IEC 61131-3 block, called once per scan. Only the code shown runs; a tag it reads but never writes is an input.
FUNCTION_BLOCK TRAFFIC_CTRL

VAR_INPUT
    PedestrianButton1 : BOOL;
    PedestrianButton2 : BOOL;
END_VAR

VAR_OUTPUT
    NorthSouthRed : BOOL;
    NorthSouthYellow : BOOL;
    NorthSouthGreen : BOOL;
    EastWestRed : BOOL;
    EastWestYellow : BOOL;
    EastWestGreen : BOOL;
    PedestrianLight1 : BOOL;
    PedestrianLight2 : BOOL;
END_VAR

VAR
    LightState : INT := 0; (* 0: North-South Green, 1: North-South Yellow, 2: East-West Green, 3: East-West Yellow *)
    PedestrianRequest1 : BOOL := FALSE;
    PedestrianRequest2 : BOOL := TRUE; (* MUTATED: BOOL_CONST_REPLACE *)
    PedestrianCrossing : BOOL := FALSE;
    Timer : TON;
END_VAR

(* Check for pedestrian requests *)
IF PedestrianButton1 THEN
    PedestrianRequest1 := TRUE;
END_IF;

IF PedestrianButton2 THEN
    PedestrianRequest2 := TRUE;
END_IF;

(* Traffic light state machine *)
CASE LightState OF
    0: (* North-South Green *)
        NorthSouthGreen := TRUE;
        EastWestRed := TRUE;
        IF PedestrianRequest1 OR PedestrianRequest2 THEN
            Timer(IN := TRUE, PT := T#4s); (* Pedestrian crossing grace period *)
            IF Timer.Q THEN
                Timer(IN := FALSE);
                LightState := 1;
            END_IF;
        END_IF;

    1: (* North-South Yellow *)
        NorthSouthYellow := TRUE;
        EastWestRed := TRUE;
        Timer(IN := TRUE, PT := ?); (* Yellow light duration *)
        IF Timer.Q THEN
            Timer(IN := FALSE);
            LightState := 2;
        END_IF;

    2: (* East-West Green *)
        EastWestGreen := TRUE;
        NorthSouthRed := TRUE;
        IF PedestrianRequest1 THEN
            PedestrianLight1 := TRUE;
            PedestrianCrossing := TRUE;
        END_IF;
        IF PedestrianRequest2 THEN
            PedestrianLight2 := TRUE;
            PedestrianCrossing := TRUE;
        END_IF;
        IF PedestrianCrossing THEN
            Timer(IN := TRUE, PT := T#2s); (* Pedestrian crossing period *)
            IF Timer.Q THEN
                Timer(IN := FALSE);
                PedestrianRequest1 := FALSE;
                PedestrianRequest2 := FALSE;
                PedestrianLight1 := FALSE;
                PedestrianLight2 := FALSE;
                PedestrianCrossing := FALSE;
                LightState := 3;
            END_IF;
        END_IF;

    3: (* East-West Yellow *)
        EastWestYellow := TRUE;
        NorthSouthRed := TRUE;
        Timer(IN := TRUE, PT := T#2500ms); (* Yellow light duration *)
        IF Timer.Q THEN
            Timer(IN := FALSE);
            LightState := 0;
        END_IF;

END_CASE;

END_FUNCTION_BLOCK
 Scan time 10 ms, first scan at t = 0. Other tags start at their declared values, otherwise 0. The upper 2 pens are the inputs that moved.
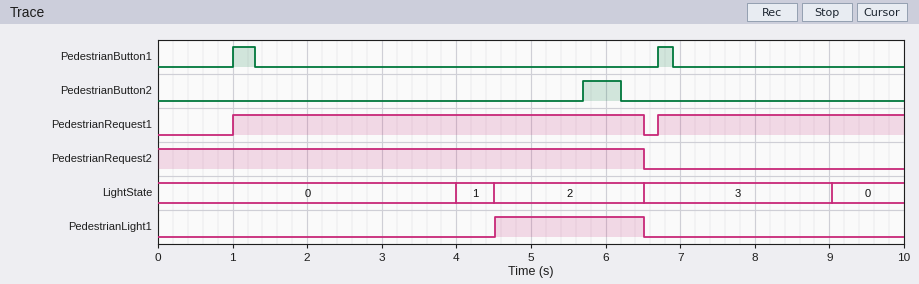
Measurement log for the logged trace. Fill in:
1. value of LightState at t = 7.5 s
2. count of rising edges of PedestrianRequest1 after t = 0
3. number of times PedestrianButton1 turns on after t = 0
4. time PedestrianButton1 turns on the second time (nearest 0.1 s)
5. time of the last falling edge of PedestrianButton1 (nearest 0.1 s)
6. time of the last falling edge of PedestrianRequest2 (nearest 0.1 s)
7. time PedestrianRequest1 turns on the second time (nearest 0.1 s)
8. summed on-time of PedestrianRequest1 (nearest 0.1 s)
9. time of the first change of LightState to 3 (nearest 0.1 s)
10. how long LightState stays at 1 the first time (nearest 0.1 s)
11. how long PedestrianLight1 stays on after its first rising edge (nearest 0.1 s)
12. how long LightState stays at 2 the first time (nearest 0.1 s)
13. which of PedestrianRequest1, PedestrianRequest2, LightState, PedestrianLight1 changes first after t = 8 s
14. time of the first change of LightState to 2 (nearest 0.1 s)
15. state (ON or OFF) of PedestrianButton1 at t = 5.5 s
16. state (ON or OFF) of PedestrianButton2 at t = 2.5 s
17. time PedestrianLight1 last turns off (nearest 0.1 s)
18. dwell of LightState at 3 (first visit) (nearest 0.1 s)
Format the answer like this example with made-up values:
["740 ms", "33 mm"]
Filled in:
["3", "2", "2", "6.7 s", "6.9 s", "6.5 s", "6.7 s", "8.8 s", "6.5 s", "0.5 s", "2.0 s", "2.0 s", "LightState", "4.5 s", "OFF", "OFF", "6.5 s", "2.5 s"]
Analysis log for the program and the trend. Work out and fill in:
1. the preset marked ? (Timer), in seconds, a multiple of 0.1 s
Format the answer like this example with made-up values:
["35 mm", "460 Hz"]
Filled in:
["0.5 s"]
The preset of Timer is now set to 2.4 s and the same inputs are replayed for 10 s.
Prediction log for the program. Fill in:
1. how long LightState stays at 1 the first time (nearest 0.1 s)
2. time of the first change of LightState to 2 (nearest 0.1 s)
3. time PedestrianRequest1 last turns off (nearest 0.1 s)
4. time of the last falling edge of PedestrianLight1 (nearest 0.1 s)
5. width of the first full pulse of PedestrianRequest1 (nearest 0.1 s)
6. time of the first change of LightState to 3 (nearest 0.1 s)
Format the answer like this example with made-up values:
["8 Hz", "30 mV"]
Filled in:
["2.4 s", "6.4 s", "8.4 s", "8.4 s", "7.4 s", "8.4 s"]
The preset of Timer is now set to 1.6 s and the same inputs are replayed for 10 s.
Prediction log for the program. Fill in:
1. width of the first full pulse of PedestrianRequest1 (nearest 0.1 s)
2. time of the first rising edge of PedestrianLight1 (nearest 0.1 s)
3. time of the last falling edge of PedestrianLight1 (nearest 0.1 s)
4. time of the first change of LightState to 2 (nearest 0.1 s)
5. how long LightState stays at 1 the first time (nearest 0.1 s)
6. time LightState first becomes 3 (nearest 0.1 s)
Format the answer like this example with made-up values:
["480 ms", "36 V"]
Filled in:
["6.6 s", "5.6 s", "7.6 s", "5.6 s", "1.6 s", "7.6 s"]
